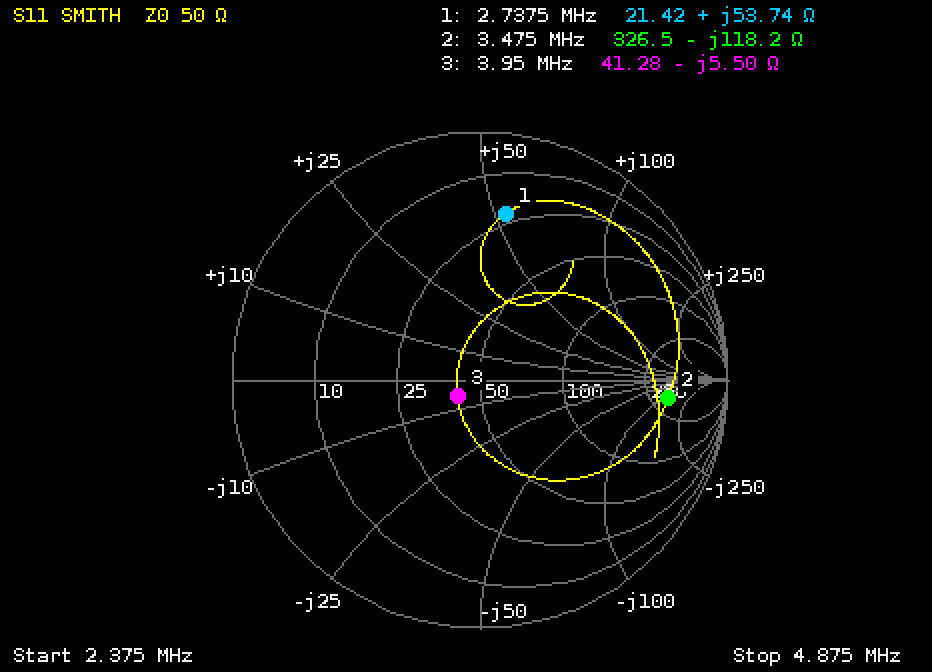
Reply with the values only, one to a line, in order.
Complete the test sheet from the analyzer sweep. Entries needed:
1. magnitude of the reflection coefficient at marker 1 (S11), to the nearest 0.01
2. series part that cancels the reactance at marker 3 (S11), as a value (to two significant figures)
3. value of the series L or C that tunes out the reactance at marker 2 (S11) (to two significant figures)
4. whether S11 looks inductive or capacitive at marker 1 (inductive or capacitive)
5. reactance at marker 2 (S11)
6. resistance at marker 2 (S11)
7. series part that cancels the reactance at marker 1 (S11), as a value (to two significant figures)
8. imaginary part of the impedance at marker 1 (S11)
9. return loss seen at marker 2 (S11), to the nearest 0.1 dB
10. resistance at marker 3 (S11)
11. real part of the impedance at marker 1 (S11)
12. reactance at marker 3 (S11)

0.68
220 nH
5.4 µH
inductive
-118.2 Ω
326.5 Ω
1.1 nF
+53.74 Ω
2.4 dB
41.28 Ω
21.42 Ω
-5.50 Ω
